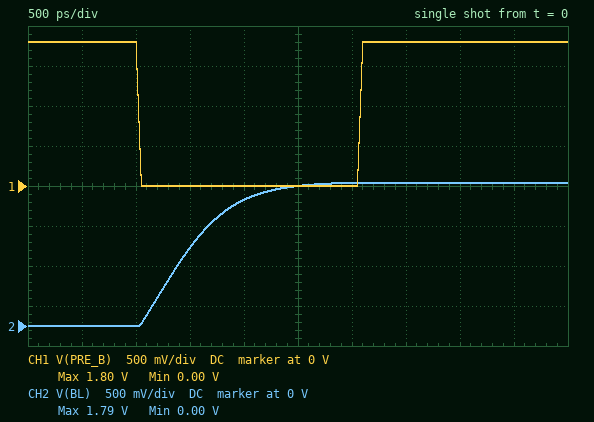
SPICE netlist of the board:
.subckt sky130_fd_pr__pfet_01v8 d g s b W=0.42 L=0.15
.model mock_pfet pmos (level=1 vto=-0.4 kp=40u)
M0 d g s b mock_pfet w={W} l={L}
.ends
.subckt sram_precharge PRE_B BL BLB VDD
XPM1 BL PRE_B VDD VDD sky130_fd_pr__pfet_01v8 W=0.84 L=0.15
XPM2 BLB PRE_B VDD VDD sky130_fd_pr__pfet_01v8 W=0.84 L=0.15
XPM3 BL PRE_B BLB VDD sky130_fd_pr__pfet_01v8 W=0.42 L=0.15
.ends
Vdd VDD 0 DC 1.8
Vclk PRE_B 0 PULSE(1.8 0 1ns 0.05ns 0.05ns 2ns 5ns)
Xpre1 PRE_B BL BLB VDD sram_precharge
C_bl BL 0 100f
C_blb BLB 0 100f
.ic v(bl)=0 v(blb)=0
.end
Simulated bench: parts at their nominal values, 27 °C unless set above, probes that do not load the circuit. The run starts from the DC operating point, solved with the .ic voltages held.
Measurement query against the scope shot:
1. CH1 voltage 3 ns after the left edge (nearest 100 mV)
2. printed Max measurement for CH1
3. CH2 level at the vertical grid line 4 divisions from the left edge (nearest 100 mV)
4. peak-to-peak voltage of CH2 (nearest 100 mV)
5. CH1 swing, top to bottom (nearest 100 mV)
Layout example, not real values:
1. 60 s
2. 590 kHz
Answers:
1. 0 V
2. 1.80 V
3. 1.6 V
4. 1.8 V
5. 1.8 V
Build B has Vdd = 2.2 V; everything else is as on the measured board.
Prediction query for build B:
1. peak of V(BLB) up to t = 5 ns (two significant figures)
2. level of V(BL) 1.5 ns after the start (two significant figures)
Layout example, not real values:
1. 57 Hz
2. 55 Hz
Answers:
1. 2.2 V
2. 1.5 V
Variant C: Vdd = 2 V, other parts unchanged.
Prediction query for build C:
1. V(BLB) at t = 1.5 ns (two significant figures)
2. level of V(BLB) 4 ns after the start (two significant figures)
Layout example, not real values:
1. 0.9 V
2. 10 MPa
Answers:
1. 1.2 V
2. 2.0 V
